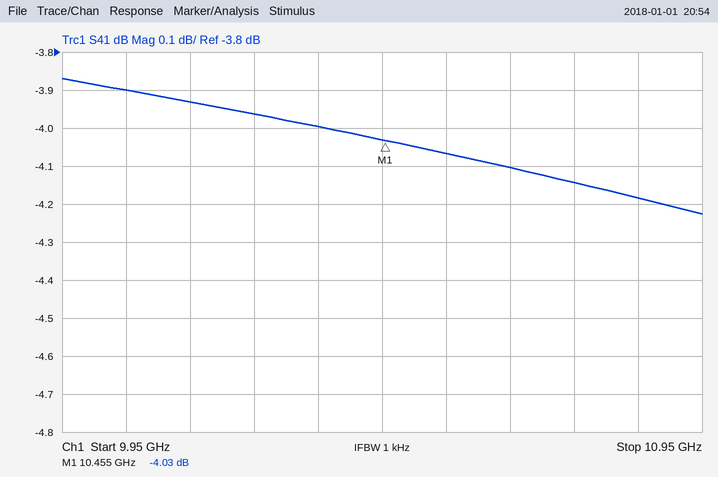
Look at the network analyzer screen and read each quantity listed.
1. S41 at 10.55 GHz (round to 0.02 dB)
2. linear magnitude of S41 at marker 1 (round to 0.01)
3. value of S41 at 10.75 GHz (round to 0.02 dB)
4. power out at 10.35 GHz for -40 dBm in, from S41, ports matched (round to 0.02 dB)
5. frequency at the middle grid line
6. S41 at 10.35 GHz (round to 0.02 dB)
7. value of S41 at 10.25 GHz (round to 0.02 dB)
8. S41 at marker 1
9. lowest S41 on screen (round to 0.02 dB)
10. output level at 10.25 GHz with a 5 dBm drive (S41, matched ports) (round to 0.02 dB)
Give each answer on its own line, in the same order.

-4.06 dB
0.63
-4.14 dB
-44.00 dBm
10.45 GHz
-4.00 dB
-3.96 dB
-4.03 dB
-4.22 dB
1.04 dBm
